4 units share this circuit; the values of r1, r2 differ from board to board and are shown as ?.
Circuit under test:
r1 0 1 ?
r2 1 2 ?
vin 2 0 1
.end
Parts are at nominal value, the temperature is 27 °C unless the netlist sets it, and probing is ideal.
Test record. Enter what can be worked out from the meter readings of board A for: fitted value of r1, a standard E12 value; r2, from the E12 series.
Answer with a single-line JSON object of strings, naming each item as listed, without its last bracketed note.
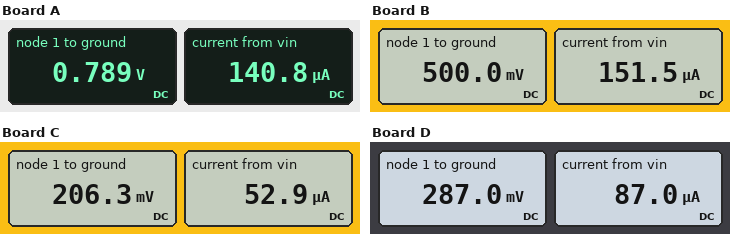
{"fitted value of r1, a standard E12 value": "5.6 kΩ", "r2, from the E12 series": "1.5 kΩ"}
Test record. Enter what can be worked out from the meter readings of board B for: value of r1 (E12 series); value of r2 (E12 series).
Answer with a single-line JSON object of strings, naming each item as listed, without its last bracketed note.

{"value of r1": "3.3 kΩ", "value of r2": "3.3 kΩ"}
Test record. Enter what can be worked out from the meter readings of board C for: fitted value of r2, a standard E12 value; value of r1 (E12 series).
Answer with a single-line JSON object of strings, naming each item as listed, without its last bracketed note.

{"fitted value of r2, a standard E12 value": "15 kΩ", "value of r1": "3.9 kΩ"}
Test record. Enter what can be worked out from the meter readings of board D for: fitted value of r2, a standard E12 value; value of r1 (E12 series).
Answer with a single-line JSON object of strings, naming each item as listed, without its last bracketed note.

{"fitted value of r2, a standard E12 value": "8.2 kΩ", "value of r1": "3.3 kΩ"}
